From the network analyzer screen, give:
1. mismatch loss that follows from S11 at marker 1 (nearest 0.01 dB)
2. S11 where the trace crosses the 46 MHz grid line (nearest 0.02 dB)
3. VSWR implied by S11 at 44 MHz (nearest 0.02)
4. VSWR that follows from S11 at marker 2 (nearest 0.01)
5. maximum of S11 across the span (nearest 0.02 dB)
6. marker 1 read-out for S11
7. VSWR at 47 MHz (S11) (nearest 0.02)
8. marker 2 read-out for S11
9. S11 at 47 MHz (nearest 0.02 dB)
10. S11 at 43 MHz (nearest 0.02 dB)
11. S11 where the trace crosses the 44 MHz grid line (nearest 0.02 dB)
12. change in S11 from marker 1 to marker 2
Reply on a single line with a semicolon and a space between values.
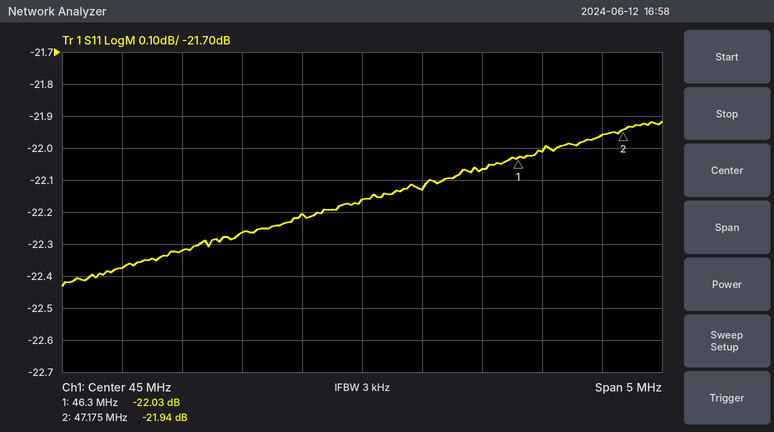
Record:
0.03 dB; -22.06 dB; 1.16; 1.17; -21.92 dB; -22.03 dB; 1.18; -21.94 dB; -21.96 dB; -22.38 dB; -22.26 dB; 0.09 dB
